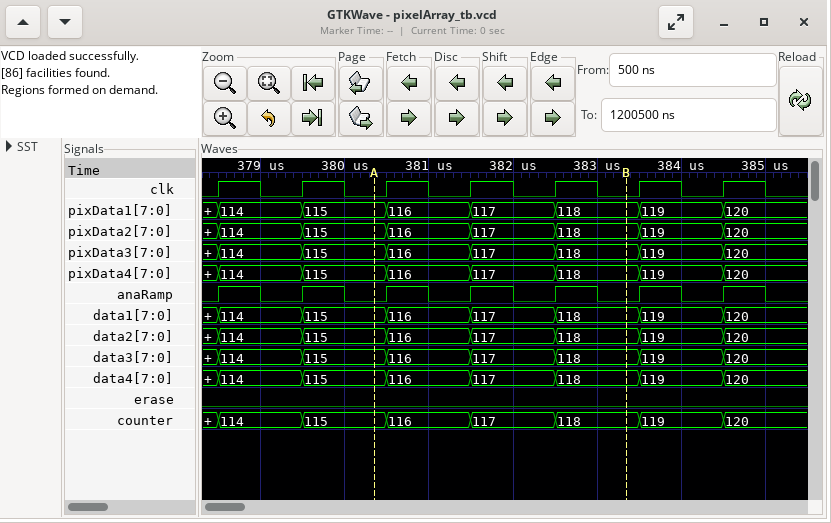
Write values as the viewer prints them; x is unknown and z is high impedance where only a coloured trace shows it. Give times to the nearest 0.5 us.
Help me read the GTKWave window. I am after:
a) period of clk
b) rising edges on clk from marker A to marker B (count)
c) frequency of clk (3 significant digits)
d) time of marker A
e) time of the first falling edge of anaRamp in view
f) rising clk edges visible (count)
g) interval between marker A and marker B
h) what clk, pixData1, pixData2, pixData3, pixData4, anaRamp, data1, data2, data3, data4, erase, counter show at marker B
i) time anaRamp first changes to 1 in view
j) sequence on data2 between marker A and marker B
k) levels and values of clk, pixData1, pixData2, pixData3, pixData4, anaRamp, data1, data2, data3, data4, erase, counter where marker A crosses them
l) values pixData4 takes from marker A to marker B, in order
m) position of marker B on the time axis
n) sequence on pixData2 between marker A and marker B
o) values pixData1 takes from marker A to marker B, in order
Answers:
1 us
3
1.00 MHz
380.5 us
379 us
7
3 us
clk=0, pixData1=118, pixData2=118, pixData3=118, pixData4=118, anaRamp=0, data1=118, data2=118, data3=118, data4=118, erase=0, counter=118
378.5 us
115, 116, 117, 118
clk=0, pixData1=115, pixData2=115, pixData3=115, pixData4=115, anaRamp=0, data1=115, data2=115, data3=115, data4=115, erase=0, counter=115
115, 116, 117, 118
383.5 us
115, 116, 117, 118
115, 116, 117, 118
